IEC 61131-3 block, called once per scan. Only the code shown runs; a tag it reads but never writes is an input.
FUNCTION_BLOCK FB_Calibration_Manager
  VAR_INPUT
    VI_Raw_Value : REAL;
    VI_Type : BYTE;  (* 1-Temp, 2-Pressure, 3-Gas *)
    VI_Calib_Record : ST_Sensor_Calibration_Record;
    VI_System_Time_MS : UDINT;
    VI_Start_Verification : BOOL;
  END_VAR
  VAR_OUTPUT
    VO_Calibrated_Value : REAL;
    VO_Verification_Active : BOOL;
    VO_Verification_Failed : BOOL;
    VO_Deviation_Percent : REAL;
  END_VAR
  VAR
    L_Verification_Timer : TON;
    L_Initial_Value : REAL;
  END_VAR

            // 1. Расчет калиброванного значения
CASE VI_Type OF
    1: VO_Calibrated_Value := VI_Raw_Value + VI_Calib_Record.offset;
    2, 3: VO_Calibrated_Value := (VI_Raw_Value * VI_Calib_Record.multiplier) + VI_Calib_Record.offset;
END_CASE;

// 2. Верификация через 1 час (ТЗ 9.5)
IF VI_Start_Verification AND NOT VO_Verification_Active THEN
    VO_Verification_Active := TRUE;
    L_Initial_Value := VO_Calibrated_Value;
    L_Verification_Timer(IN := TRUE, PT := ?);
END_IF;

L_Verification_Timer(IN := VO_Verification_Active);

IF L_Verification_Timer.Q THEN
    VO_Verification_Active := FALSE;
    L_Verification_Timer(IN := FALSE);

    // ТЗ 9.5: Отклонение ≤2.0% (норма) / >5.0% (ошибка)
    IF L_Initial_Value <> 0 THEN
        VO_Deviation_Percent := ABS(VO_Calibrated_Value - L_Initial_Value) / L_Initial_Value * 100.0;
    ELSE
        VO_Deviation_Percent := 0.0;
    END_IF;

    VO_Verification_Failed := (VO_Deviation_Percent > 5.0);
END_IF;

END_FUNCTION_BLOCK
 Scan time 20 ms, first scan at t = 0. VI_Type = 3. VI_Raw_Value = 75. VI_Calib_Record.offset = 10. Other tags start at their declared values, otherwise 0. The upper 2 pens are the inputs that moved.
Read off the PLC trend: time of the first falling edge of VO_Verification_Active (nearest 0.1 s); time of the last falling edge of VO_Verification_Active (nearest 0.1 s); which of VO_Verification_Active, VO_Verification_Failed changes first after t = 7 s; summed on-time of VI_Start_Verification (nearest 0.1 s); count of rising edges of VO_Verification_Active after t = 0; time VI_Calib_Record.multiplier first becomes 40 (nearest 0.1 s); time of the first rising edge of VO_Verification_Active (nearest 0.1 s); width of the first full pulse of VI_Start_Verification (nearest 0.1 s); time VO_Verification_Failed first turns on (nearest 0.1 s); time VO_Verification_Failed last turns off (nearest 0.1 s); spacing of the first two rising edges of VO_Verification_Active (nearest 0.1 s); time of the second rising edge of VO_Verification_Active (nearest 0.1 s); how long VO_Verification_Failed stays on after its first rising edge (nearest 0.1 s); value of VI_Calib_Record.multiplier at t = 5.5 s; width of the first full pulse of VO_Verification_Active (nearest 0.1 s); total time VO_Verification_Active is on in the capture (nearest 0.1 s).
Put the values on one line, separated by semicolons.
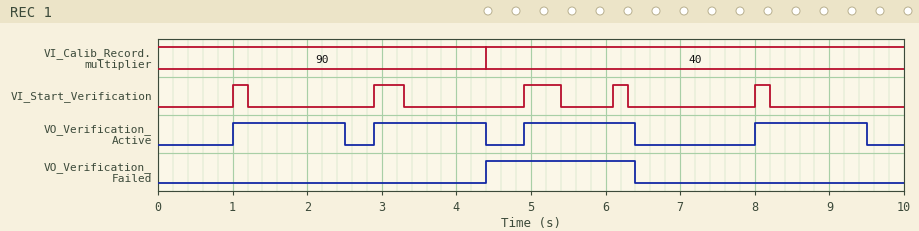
2.5 s; 9.5 s; VO_Verification_Active; 1.5 s; 4; 4.4 s; 1.0 s; 0.2 s; 4.4 s; 6.4 s; 1.9 s; 2.9 s; 2.0 s; 40; 1.5 s; 6.0 s
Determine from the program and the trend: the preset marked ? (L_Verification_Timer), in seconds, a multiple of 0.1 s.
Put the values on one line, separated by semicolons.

1.5 s
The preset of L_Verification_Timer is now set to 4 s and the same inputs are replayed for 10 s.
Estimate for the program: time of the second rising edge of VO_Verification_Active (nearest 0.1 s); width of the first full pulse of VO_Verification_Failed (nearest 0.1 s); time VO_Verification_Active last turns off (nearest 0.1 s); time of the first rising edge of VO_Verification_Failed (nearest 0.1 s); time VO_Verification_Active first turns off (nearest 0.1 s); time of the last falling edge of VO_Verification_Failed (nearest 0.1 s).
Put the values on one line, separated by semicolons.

5.0 s; 4.0 s; 9.0 s; 5.0 s; 5.0 s; 9.0 s
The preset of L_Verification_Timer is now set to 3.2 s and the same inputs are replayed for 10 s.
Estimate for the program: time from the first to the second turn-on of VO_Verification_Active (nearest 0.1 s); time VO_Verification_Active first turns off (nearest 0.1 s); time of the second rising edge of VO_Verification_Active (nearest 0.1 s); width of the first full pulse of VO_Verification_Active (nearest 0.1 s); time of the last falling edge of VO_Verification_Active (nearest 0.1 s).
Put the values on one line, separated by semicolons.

3.9 s; 4.2 s; 4.9 s; 3.2 s; 8.1 s
